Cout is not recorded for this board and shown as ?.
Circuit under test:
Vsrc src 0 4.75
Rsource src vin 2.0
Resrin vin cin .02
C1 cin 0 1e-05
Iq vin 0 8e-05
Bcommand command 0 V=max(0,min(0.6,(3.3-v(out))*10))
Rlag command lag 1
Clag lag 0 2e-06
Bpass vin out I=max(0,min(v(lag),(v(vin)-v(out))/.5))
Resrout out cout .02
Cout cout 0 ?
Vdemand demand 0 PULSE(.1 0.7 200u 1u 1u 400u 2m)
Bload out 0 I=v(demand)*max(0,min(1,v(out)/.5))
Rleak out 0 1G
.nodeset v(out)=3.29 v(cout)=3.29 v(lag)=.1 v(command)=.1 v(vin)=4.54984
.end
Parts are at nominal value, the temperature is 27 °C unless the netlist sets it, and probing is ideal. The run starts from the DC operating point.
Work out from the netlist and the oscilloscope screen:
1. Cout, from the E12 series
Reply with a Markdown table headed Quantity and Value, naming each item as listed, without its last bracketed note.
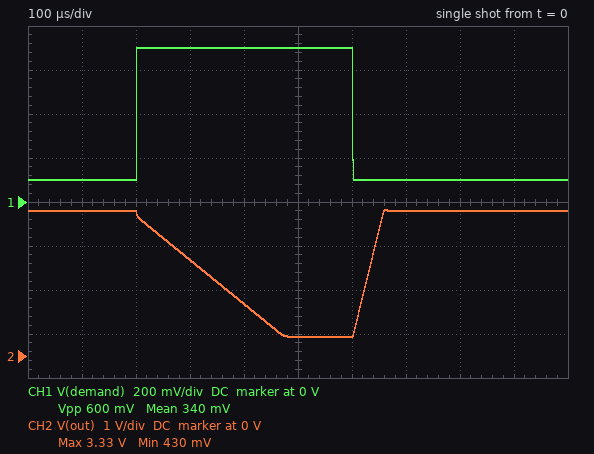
| Quantity | Value |
|---|---|
| Cout, from the E12 series | 10 µF |
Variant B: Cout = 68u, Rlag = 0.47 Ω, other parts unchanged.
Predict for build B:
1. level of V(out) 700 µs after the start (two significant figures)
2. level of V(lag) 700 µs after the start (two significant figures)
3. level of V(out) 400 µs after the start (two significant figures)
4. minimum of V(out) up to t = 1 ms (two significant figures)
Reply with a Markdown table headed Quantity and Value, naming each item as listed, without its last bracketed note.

| Quantity | Value |
|---|---|
| level of V(out) 700 µs after the start | 3.3 V |
| level of V(lag) 700 µs after the start | 130 mV |
| level of V(out) 400 µs after the start | 3.0 V |
| minimum of V(out) up to t = 1 ms | 2.7 V |
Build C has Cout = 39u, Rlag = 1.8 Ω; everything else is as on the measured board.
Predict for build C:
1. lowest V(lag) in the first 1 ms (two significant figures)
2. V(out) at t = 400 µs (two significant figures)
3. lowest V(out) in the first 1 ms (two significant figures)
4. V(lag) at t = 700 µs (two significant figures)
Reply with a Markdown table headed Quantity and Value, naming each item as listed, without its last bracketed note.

| Quantity | Value |
|---|---|
| lowest V(lag) in the first 1 ms | 59 mV |
| V(out) at t = 400 µs | 2.7 V |
| lowest V(out) in the first 1 ms | 2.2 V |
| V(lag) at t = 700 µs | 69 mV |
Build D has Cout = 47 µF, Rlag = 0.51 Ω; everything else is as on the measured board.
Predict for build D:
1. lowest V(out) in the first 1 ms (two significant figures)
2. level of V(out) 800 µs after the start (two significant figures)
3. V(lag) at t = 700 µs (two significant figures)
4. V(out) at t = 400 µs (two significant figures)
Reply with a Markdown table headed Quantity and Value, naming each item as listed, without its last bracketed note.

| Quantity | Value |
|---|---|
| lowest V(out) in the first 1 ms | 2.4 V |
| level of V(out) 800 µs after the start | 3.3 V |
| V(lag) at t = 700 µs | 110 mV |
| V(out) at t = 400 µs | 2.8 V |
